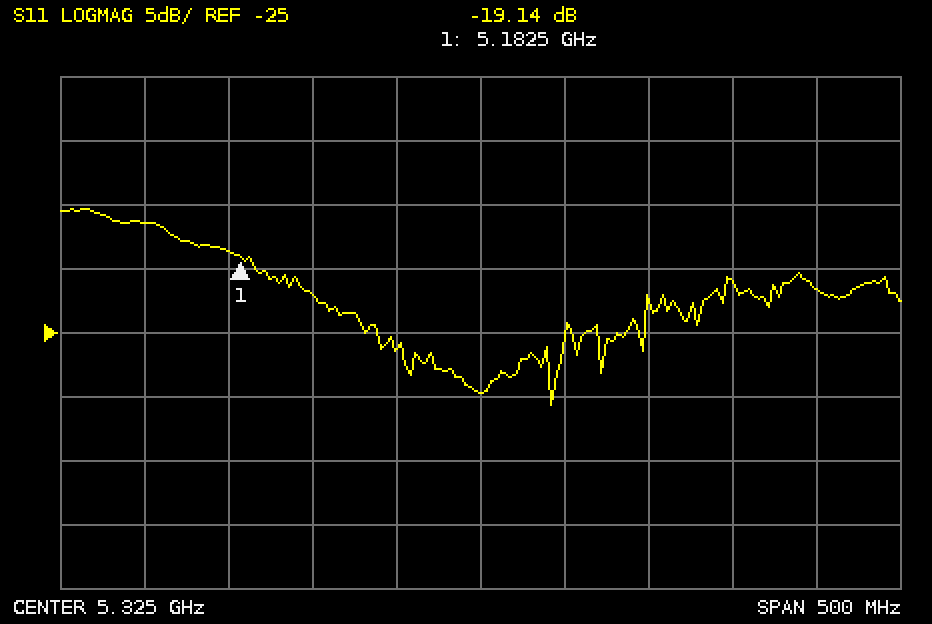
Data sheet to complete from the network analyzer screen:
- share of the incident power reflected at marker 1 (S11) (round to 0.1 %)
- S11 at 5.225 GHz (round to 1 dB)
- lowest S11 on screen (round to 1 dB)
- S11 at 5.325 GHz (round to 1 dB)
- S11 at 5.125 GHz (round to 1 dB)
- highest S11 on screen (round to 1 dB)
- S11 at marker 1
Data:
1.2 %
-22 dB
-31 dB
-30 dB
-16 dB
-15 dB
-19.14 dB
